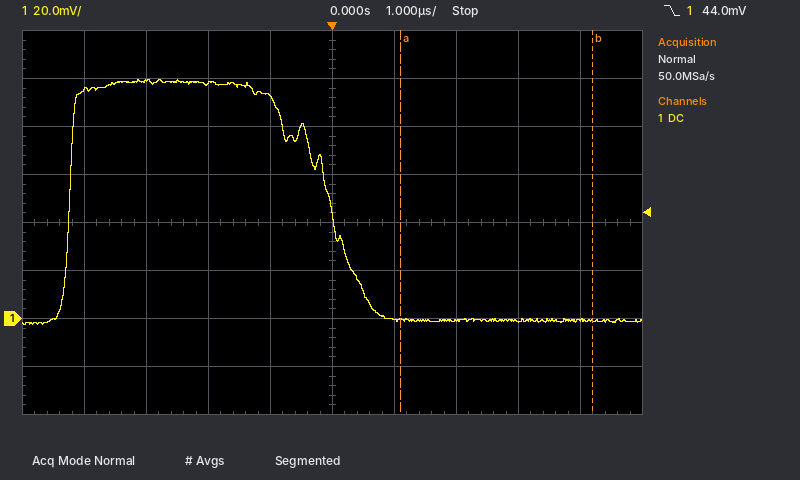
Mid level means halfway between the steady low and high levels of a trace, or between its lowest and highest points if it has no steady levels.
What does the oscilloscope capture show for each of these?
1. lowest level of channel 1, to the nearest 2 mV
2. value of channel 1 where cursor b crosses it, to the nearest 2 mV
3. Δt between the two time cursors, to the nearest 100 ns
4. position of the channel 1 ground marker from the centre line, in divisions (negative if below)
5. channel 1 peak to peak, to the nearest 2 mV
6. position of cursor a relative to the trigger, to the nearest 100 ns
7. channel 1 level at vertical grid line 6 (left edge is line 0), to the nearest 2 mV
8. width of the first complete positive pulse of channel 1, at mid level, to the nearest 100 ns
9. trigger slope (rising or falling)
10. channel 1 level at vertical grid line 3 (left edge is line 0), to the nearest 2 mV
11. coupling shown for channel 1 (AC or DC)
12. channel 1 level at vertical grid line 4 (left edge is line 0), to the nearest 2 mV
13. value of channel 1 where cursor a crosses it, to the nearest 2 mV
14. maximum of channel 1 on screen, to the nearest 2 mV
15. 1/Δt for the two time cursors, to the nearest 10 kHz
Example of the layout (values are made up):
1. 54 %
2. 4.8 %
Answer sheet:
1. -2 mV
2. 0 mV
3. 3.1 µs
4. -2.0 div
5. 102 mV
6. +1.1 µs
7. 0 mV
8. 4.2 µs
9. falling
10. 98 mV
11. DC
12. 92 mV
13. 0 mV
14. 100 mV
15. 320 kHz
